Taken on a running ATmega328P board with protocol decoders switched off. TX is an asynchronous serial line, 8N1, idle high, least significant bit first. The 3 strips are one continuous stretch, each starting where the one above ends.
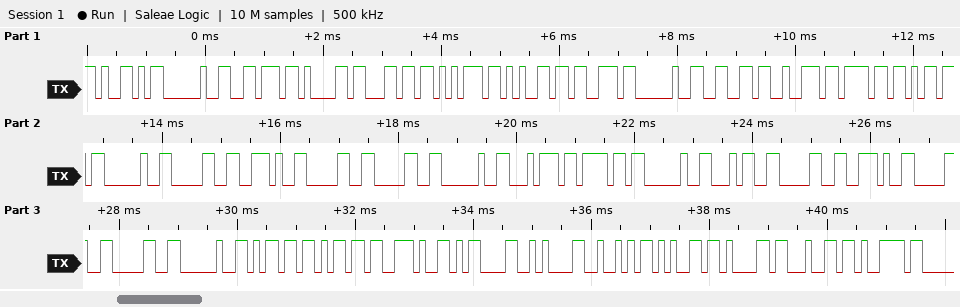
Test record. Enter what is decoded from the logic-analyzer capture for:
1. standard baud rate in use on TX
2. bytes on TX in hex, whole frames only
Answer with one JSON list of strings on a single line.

["9600 baud", "59 20 76 61 6C 75 65 73 20 66 72 6F 6D 20 30 2E 30 30 20 74 6F 20 34 30 2E 30 30 20 6D 6D 2E 0D 0A 52 65 61 64 79"]
